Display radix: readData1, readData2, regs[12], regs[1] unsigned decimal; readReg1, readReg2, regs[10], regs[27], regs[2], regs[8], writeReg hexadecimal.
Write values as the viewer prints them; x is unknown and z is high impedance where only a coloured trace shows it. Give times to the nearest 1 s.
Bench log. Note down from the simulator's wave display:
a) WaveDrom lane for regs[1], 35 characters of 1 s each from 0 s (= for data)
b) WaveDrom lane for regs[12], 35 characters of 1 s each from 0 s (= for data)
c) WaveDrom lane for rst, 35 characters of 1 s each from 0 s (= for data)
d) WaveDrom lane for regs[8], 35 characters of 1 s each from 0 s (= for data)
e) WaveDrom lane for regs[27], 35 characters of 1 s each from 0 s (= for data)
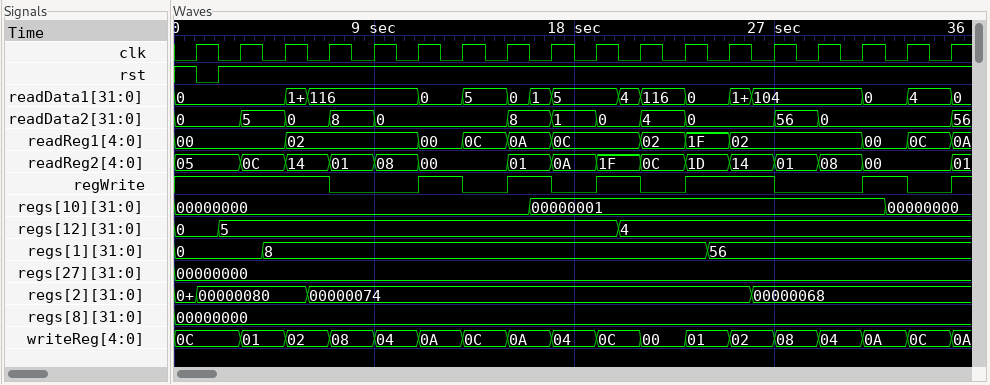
{name: 'regs[1]', wave: '=...=...................=..........', data: '0 8 56'}
{name: 'regs[12]', wave: '=.=.................=..............', data: '0 5 4'}
{name: 'rst', wave: '101................................'}
{name: 'regs[8]', wave: '=..................................', data: '00000000'}
{name: 'regs[27]', wave: '=..................................', data: '00000000'}
